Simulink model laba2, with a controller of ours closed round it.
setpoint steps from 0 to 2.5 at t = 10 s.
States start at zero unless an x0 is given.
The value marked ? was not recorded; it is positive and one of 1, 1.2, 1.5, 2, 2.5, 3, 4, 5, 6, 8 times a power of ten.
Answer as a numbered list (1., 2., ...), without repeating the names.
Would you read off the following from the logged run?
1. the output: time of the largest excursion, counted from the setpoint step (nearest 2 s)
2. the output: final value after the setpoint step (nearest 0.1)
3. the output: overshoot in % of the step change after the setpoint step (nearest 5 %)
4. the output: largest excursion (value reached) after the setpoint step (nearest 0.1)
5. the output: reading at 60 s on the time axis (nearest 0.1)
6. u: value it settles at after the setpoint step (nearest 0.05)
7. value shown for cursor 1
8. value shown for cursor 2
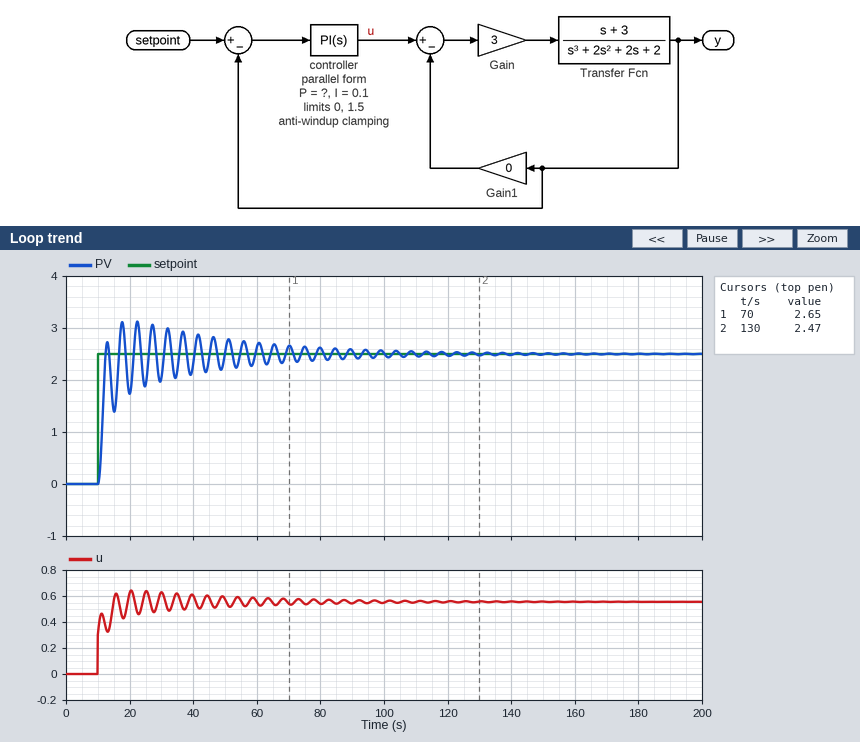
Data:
1. 12 s
2. 2.5
3. 25 %
4. 3.1
5. 2.6
6. 0.55
7. 2.65
8. 2.47
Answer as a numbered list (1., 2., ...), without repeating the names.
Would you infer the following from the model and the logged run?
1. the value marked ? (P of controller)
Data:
1. 0.12
